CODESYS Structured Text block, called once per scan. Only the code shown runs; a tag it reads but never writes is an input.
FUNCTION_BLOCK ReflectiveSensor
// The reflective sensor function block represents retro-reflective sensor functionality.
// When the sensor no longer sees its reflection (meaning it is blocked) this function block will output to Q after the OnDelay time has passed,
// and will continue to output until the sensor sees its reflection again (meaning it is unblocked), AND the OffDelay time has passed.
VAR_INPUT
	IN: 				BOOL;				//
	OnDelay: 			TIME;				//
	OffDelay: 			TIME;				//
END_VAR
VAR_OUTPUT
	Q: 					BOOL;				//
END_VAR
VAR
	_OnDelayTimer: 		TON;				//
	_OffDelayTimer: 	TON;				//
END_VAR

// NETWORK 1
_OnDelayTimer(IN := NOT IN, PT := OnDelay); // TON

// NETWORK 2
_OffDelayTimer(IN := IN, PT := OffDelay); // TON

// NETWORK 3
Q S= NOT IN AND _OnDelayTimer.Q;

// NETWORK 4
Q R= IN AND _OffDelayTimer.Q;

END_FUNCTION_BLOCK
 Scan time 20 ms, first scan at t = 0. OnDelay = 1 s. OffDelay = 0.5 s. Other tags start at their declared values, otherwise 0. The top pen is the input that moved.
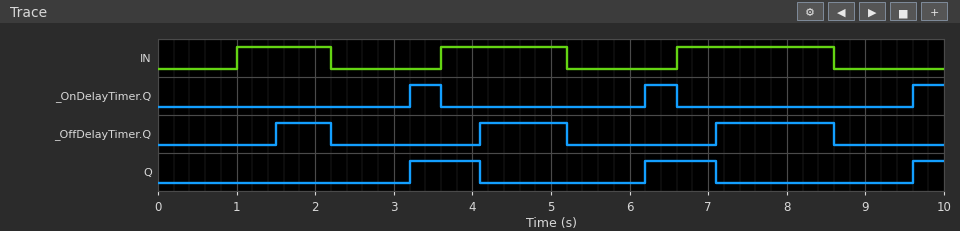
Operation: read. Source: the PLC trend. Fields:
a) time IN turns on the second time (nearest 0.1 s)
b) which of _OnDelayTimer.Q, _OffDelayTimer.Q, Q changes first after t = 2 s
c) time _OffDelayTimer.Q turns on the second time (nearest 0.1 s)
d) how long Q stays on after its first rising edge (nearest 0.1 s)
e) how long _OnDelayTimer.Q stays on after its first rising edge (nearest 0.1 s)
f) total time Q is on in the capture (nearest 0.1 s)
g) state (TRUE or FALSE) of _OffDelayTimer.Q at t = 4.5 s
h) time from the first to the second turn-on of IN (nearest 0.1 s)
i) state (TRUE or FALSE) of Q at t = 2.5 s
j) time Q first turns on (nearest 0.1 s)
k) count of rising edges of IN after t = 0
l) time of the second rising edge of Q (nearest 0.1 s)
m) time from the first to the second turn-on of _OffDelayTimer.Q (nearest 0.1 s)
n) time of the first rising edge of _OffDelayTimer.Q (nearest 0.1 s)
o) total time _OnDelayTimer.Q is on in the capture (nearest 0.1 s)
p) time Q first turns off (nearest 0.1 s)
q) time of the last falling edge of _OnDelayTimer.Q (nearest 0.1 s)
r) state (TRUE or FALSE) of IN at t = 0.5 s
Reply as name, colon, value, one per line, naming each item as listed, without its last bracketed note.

time IN turns on the second time: 3.6 s
which of _OnDelayTimer.Q, _OffDelayTimer.Q, Q changes first after t = 2 s: _OffDelayTimer.Q
time _OffDelayTimer.Q turns on the second time: 4.1 s
how long Q stays on after its first rising edge: 0.9 s
how long _OnDelayTimer.Q stays on after its first rising edge: 0.4 s
total time Q is on in the capture: 2.2 s
state (TRUE or FALSE) of _OffDelayTimer.Q at t = 4.5 s: TRUE
time from the first to the second turn-on of IN: 2.6 s
state (TRUE or FALSE) of Q at t = 2.5 s: FALSE
time Q first turns on: 3.2 s
count of rising edges of IN after t = 0: 3
time of the second rising edge of Q: 6.2 s
time from the first to the second turn-on of _OffDelayTimer.Q: 2.6 s
time of the first rising edge of _OffDelayTimer.Q: 1.5 s
total time _OnDelayTimer.Q is on in the capture: 1.2 s
time Q first turns off: 4.1 s
time of the last falling edge of _OnDelayTimer.Q: 6.6 s
state (TRUE or FALSE) of IN at t = 0.5 s: FALSE
